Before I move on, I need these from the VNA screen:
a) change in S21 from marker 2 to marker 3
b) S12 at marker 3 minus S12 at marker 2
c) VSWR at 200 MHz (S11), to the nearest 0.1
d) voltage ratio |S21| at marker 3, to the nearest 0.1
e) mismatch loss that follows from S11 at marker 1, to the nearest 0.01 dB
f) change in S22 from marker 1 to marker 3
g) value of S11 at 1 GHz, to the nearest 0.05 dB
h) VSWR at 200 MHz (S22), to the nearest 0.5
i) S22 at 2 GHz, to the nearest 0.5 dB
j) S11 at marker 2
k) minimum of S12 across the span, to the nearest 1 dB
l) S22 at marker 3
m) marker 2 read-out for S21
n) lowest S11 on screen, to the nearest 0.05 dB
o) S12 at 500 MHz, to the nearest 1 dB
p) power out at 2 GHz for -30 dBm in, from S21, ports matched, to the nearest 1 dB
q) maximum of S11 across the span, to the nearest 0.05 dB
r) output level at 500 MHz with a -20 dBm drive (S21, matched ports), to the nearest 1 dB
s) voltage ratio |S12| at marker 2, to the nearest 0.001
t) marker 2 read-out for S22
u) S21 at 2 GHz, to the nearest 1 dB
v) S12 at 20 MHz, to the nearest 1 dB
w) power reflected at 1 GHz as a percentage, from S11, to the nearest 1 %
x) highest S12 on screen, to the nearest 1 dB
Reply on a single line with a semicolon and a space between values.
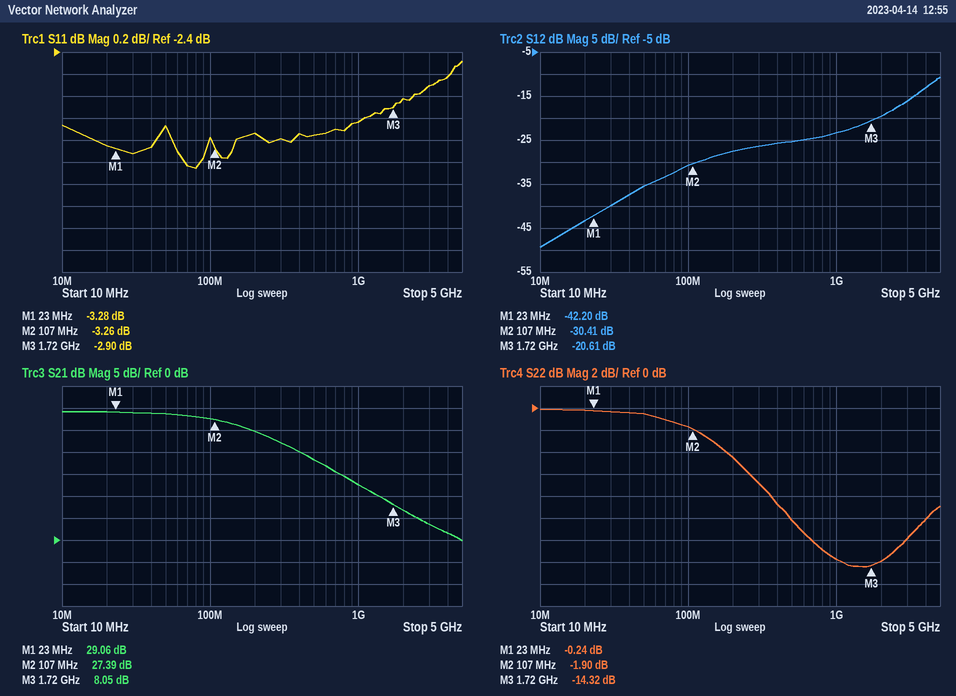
-19.34 dB; 9.80 dB; 5.6; 2.5; 2.76 dB; -14.08 dB; -3.05 dB; 4.0; -14.0 dB; -3.26 dB; -49 dB; -14.32 dB; 27.39 dB; -3.45 dB; -25 dB; -23 dBm; -2.50 dB; -2 dBm; 0.030; -1.90 dB; 7 dB; -43 dB; 50 %; -11 dB
